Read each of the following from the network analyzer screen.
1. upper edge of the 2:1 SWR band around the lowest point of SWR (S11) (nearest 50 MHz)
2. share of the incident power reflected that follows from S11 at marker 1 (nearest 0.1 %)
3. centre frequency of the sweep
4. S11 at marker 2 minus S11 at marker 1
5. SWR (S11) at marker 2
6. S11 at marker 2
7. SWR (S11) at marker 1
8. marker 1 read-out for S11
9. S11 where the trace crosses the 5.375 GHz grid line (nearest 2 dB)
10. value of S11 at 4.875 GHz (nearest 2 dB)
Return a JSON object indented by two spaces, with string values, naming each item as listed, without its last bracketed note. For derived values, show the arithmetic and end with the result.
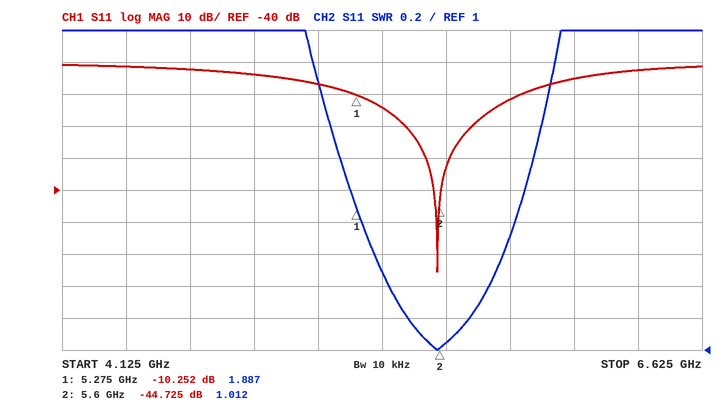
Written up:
{
  "upper edge of the 2:1 SWR band around the lowest point of SWR (S11)": "5.95 GHz",
  "share of the incident power reflected that follows from S11 at marker 1": "10^(-10.252/10) ≈ 9.4 %",
  "centre frequency of the sweep": "5.375 GHz",
  "S11 at marker 2 minus S11 at marker 1": "-44.725 − (-10.252) = -34.473 dB",
  "SWR (S11) at marker 2": "1.012",
  "S11 at marker 2": "-44.725 dB",
  "SWR (S11) at marker 1": "1.887",
  "marker 1 read-out for S11": "-10.252 dB",
  "S11 where the trace crosses the 5.375 GHz grid line": "-14 dB",
  "value of S11 at 4.875 GHz": "-4 dB"
}
